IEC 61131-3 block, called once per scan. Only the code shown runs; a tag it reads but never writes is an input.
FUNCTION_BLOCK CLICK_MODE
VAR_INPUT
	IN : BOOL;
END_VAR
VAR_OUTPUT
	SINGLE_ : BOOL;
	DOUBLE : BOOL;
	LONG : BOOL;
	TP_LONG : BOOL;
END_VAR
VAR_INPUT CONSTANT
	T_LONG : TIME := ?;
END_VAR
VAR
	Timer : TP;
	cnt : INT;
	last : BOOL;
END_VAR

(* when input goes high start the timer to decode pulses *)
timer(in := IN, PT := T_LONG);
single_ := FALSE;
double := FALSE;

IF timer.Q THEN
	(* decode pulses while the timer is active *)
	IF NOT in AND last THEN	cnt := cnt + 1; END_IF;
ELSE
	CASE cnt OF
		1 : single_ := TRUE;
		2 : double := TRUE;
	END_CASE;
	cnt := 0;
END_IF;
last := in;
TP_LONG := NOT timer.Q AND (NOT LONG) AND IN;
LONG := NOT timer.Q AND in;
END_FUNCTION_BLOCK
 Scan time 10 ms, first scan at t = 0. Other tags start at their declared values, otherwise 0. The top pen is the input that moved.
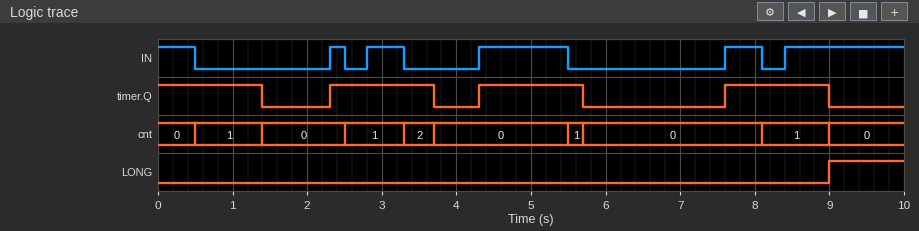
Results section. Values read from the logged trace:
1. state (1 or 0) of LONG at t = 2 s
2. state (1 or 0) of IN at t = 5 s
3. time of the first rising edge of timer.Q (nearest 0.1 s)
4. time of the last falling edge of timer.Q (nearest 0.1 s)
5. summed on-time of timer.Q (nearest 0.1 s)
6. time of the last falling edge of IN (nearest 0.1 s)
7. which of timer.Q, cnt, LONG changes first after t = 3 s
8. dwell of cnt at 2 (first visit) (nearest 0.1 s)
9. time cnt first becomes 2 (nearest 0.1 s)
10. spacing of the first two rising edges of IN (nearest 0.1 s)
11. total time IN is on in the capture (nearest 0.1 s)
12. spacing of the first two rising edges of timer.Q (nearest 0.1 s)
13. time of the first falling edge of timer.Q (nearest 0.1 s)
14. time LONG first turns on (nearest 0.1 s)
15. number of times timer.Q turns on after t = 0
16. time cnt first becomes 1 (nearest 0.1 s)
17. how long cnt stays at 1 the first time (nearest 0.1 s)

0
1
2.3 s
9.0 s
5.6 s
8.1 s
cnt
0.4 s
3.3 s
0.5 s
4.5 s
2.0 s
1.4 s
9.0 s
3
0.5 s
0.9 s
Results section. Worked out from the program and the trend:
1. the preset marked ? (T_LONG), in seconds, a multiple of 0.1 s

1.4 s
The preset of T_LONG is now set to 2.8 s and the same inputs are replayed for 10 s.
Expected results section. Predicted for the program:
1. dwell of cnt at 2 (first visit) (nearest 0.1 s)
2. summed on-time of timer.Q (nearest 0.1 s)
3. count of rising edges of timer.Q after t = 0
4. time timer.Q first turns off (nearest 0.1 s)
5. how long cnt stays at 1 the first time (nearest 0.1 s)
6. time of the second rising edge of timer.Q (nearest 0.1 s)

0.3 s
8.0 s
2
2.8 s
2.0 s
7.6 s
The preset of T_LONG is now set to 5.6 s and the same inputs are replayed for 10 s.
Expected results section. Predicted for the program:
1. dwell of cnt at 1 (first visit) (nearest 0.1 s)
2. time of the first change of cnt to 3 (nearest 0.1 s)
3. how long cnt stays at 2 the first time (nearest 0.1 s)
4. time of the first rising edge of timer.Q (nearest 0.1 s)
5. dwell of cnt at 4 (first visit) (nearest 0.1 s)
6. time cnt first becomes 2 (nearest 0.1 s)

2.0 s
3.3 s
0.8 s
7.6 s
0.1 s
2.5 s
